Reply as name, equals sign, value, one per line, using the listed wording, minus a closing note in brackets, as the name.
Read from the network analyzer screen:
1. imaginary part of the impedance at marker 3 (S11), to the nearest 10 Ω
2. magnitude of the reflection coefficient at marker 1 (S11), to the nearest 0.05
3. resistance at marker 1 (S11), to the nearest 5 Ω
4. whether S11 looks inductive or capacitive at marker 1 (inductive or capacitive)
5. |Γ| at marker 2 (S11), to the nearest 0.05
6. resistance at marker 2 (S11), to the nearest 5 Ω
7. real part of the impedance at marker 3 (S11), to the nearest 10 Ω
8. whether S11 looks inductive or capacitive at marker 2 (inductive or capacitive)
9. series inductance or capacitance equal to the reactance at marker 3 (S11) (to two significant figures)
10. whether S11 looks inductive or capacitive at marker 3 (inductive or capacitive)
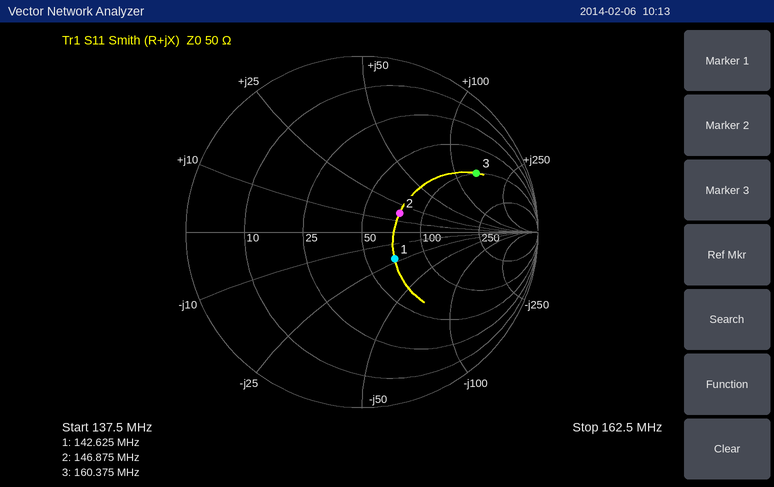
imaginary part of the impedance at marker 3 (S11), to the nearest 10 Ω = +140 Ω
magnitude of the reflection coefficient at marker 1 (S11), to the nearest 0.05 = 0.25
resistance at marker 1 (S11), to the nearest 5 Ω = 70 Ω
whether S11 looks inductive or capacitive at marker 1 = capacitive
|Γ| at marker 2 (S11), to the nearest 0.05 = 0.25
resistance at marker 2 (S11), to the nearest 5 Ω = 75 Ω
real part of the impedance at marker 3 (S11), to the nearest 10 Ω = 100 Ω
whether S11 looks inductive or capacitive at marker 2 = inductive
series inductance or capacitance equal to the reactance at marker 3 (S11) = 140 nH
whether S11 looks inductive or capacitive at marker 3 = inductive
